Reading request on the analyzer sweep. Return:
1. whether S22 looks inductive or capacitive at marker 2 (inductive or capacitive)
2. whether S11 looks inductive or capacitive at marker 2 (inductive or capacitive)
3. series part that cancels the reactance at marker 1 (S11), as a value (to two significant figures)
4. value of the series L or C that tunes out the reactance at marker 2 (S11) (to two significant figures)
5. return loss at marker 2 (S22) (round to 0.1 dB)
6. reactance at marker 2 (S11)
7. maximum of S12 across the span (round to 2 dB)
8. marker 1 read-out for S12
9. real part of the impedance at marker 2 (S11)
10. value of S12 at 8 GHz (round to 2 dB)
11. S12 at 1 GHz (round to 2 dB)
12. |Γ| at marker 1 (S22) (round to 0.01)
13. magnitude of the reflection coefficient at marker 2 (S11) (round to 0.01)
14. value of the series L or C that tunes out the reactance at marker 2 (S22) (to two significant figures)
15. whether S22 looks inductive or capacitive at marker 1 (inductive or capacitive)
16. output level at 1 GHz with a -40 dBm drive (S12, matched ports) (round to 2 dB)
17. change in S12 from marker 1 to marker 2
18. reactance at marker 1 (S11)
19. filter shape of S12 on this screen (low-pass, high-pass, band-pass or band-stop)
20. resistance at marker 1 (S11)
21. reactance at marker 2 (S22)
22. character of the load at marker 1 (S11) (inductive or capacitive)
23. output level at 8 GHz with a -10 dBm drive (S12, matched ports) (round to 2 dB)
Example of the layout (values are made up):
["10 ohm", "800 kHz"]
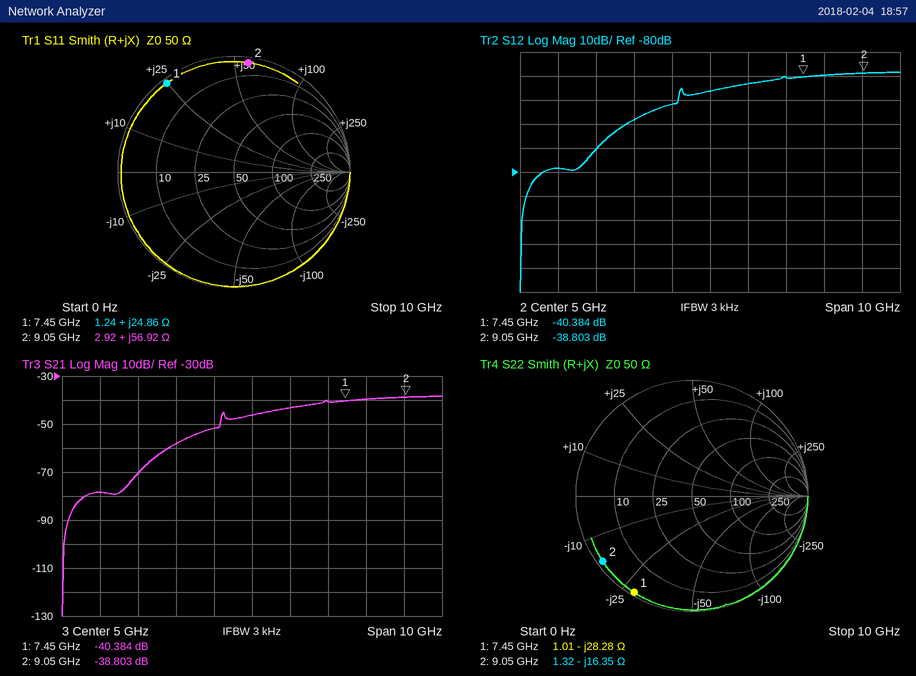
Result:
["capacitive", "inductive", "860 fF", "310 fF", "0.4 dB", "+56.92 Ω", "-38 dB", "-40.384 dB", "2.92 Ω", "-40 dB", "-78 dB", "0.97", "0.95", "290 pH", "capacitive", "-118 dBm", "1.581 dB", "+24.86 Ω", "high-pass", "1.24 Ω", "-16.35 Ω", "inductive", "-50 dBm"]
